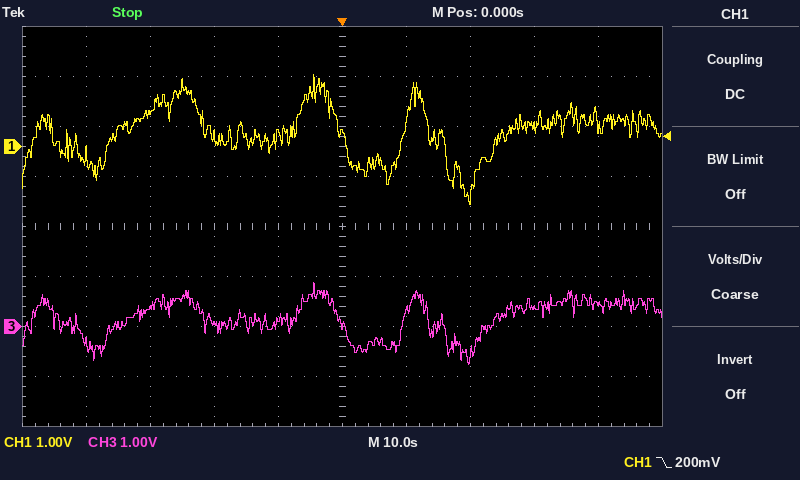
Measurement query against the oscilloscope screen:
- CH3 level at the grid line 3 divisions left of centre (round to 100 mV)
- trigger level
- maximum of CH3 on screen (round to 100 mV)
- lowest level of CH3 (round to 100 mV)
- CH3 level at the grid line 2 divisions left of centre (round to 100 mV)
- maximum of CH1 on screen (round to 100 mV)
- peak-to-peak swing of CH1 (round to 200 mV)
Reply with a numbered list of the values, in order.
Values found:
1. 400 mV
2. 200 mV
3. 900 mV
4. -800 mV
5. 100 mV
6. 1.4 V
7. 2.6 V
